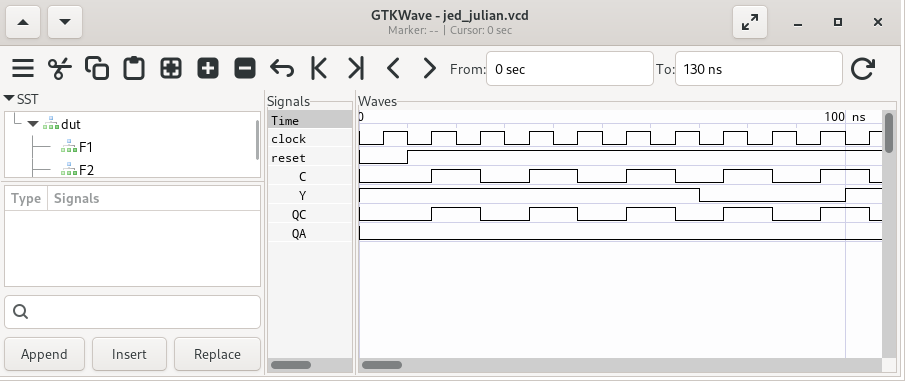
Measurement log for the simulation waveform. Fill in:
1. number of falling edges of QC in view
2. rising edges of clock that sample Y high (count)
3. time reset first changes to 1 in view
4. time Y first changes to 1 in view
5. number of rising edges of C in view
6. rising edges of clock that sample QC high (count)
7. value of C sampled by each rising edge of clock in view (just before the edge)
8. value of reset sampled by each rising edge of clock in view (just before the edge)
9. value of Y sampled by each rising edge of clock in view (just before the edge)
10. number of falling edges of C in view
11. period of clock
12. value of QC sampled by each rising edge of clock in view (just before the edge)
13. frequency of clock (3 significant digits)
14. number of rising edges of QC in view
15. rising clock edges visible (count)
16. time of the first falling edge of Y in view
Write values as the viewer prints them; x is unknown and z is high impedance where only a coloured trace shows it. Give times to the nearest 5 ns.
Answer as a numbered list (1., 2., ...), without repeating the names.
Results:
1. 5
2. 8
3. 10 ns
4. 100 ns
5. 5
6. 5
7. 0 0 1 0 1 0 1 0 1 0 1
8. 0 1 1 1 1 1 1 1 1 1 1
9. 1 1 1 1 1 1 1 0 0 0 1
10. 5
11. 10 ns
12. 0 0 1 0 1 0 1 0 1 0 1
13. 100 MHz
14. 5
15. 11
16. 70 ns
